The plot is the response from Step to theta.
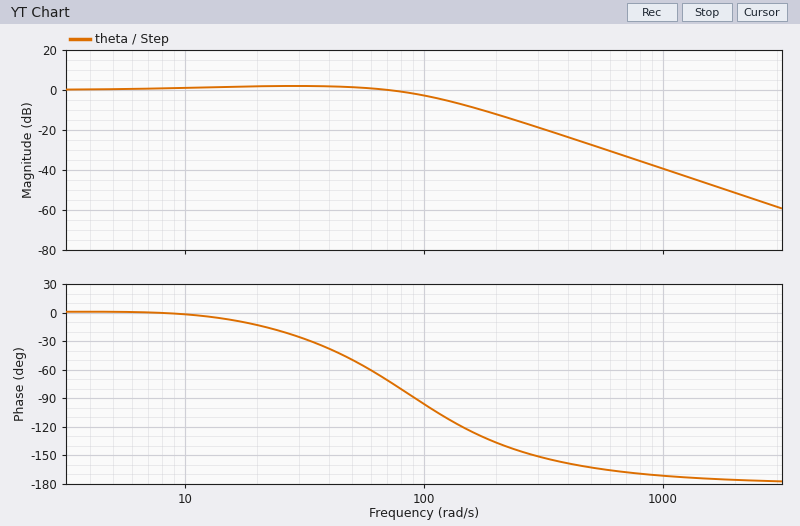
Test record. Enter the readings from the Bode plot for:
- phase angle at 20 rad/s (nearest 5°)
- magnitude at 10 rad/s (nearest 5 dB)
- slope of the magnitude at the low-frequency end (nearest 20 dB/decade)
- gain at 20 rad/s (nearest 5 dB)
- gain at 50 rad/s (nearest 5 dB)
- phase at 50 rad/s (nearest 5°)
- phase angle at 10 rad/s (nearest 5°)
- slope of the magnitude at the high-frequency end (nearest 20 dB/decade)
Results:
-15°
0 dB
0 dB/decade
0 dB
0 dB
-50°
0°
-40 dB/decade
